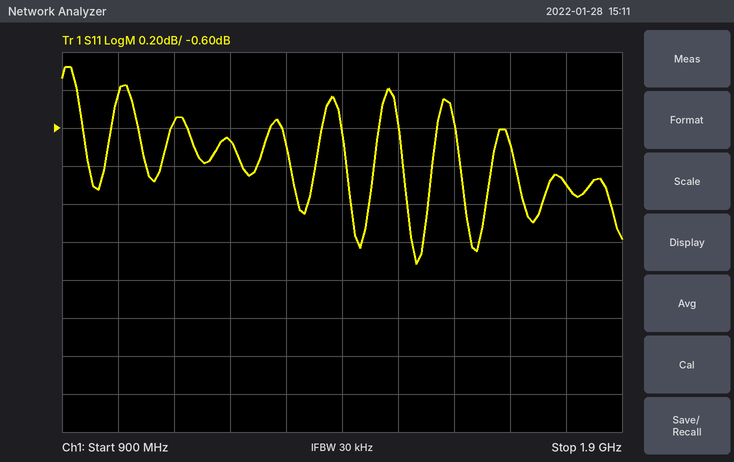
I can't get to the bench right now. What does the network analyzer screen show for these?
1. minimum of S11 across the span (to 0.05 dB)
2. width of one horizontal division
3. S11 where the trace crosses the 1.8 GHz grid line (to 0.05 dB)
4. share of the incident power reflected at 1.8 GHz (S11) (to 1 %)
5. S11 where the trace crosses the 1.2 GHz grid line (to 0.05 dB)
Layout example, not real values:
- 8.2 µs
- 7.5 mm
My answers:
- -1.30 dB
- 100 MHz
- -0.90 dB
- 81 %
- -0.65 dB
